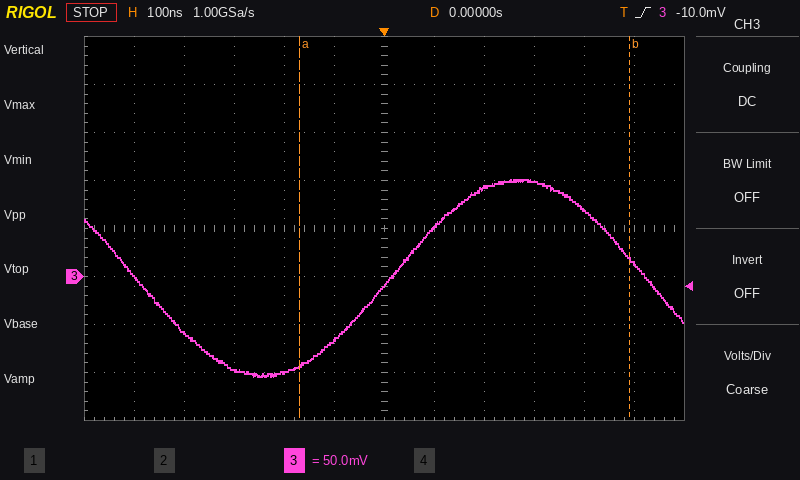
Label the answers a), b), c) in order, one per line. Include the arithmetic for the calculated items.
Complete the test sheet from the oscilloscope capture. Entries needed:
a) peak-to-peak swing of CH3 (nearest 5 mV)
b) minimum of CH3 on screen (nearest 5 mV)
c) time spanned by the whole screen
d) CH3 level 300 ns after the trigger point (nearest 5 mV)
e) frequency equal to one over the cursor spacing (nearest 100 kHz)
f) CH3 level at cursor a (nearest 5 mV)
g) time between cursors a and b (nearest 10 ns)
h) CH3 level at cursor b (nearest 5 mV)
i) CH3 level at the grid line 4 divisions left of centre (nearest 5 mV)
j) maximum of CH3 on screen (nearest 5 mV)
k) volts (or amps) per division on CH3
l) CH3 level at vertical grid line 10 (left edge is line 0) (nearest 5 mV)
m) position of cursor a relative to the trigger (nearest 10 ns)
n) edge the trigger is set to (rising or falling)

a) 100 mV − (-105 mV) = 205 mV
b) -105 mV
c) 1.2 µs
d) 100 mV
e) 1 / 660 ns ≈ 1.5 MHz
f) -90 mV
g) 660 ns
h) 20 mV
i) -60 mV
j) 100 mV
k) 50 mV
l) 70 mV
m) -170 ns
n) rising
